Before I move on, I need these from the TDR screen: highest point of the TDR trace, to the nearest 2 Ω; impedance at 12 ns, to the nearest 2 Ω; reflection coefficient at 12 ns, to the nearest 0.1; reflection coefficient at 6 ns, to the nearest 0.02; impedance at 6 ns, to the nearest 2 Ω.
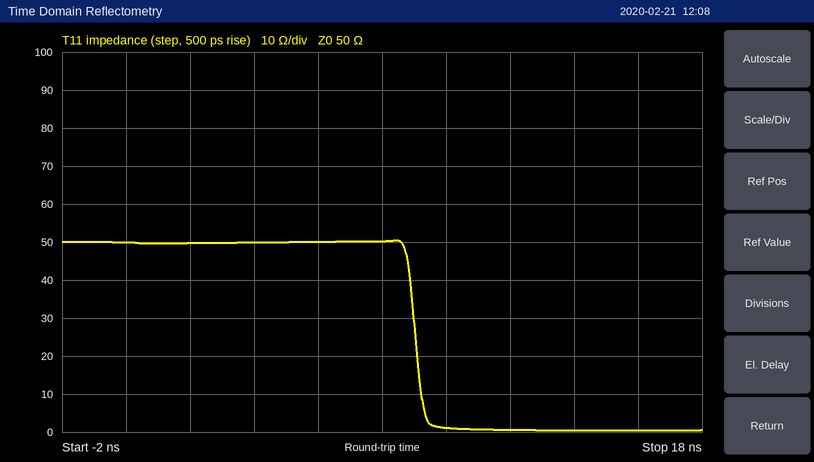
50 Ω
0 Ω
-1.0
0.00
50 Ω
